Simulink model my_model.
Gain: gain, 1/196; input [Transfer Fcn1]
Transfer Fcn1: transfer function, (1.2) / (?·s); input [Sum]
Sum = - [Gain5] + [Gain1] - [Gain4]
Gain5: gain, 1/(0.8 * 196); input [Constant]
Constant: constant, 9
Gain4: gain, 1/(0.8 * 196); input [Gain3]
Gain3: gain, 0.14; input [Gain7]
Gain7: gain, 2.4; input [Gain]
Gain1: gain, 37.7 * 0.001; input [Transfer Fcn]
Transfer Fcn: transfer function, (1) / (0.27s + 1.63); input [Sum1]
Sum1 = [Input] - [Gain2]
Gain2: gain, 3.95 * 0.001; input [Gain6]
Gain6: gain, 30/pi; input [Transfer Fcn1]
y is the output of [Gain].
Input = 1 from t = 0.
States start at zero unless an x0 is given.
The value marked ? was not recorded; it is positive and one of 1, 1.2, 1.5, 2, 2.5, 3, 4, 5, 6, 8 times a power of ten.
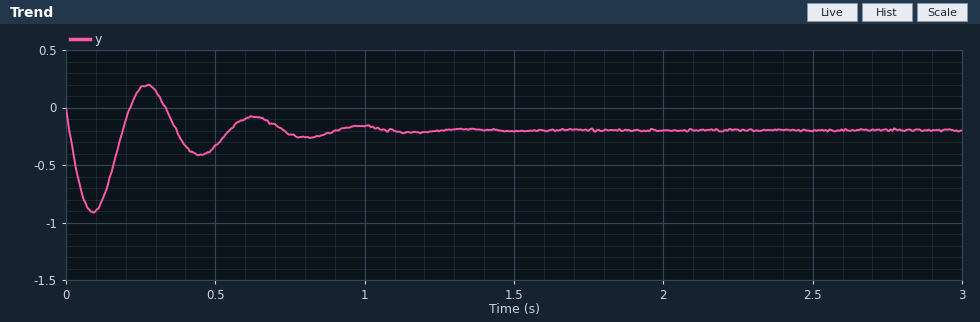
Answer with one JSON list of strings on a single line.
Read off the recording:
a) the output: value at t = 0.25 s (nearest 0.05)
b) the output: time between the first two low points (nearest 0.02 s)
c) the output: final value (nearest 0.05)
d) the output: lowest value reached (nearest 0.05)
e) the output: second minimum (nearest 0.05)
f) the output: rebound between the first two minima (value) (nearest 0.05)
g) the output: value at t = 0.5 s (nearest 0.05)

["0.15", "0.36 s", "-0.20", "-0.90", "-0.40", "0.20", "-0.35"]
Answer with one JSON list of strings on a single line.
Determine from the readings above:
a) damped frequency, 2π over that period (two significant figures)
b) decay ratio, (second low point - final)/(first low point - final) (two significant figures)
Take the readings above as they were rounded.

["17 rad/s", "0.29"]
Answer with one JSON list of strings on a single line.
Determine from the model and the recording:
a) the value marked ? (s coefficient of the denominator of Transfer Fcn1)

["2e-05"]
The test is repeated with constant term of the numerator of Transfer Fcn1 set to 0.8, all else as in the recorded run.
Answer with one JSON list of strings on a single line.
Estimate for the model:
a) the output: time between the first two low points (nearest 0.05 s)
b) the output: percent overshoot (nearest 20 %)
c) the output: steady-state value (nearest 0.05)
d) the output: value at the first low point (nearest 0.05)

["0.45 s", "280 %", "-0.20", "-0.75"]
